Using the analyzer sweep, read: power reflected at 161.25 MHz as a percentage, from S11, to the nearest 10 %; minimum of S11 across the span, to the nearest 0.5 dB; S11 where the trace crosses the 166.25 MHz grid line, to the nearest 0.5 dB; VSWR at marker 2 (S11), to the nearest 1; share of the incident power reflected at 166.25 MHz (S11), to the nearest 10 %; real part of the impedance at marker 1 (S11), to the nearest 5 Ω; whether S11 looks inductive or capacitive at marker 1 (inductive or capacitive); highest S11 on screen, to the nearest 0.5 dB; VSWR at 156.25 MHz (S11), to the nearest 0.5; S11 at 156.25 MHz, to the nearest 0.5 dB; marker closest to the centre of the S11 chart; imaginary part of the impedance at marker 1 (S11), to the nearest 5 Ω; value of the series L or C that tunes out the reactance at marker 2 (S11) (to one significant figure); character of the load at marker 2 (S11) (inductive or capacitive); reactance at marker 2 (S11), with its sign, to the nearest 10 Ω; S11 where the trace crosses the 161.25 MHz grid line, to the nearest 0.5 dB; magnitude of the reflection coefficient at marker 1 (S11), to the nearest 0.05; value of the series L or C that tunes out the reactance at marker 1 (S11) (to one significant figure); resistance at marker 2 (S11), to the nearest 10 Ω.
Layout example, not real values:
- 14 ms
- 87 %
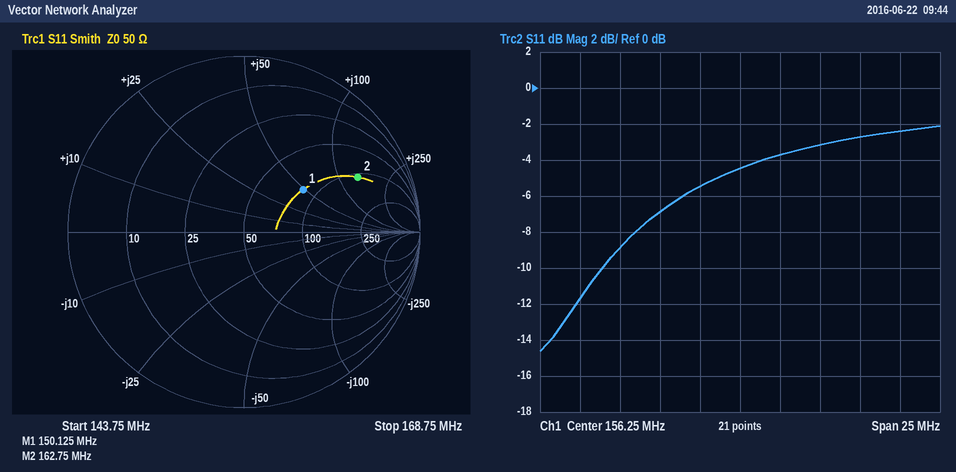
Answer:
- 50 %
- -14.5 dB
- -2.5 dB
- 6
- 60 %
- 85 Ω
- inductive
- -2.0 dB
- 4.0
- -4.5 dB
- marker 1
- +50 Ω
- 7 pF
- inductive
- +140 Ω
- -3.0 dB
- 0.40
- 20 pF
- 110 Ω
